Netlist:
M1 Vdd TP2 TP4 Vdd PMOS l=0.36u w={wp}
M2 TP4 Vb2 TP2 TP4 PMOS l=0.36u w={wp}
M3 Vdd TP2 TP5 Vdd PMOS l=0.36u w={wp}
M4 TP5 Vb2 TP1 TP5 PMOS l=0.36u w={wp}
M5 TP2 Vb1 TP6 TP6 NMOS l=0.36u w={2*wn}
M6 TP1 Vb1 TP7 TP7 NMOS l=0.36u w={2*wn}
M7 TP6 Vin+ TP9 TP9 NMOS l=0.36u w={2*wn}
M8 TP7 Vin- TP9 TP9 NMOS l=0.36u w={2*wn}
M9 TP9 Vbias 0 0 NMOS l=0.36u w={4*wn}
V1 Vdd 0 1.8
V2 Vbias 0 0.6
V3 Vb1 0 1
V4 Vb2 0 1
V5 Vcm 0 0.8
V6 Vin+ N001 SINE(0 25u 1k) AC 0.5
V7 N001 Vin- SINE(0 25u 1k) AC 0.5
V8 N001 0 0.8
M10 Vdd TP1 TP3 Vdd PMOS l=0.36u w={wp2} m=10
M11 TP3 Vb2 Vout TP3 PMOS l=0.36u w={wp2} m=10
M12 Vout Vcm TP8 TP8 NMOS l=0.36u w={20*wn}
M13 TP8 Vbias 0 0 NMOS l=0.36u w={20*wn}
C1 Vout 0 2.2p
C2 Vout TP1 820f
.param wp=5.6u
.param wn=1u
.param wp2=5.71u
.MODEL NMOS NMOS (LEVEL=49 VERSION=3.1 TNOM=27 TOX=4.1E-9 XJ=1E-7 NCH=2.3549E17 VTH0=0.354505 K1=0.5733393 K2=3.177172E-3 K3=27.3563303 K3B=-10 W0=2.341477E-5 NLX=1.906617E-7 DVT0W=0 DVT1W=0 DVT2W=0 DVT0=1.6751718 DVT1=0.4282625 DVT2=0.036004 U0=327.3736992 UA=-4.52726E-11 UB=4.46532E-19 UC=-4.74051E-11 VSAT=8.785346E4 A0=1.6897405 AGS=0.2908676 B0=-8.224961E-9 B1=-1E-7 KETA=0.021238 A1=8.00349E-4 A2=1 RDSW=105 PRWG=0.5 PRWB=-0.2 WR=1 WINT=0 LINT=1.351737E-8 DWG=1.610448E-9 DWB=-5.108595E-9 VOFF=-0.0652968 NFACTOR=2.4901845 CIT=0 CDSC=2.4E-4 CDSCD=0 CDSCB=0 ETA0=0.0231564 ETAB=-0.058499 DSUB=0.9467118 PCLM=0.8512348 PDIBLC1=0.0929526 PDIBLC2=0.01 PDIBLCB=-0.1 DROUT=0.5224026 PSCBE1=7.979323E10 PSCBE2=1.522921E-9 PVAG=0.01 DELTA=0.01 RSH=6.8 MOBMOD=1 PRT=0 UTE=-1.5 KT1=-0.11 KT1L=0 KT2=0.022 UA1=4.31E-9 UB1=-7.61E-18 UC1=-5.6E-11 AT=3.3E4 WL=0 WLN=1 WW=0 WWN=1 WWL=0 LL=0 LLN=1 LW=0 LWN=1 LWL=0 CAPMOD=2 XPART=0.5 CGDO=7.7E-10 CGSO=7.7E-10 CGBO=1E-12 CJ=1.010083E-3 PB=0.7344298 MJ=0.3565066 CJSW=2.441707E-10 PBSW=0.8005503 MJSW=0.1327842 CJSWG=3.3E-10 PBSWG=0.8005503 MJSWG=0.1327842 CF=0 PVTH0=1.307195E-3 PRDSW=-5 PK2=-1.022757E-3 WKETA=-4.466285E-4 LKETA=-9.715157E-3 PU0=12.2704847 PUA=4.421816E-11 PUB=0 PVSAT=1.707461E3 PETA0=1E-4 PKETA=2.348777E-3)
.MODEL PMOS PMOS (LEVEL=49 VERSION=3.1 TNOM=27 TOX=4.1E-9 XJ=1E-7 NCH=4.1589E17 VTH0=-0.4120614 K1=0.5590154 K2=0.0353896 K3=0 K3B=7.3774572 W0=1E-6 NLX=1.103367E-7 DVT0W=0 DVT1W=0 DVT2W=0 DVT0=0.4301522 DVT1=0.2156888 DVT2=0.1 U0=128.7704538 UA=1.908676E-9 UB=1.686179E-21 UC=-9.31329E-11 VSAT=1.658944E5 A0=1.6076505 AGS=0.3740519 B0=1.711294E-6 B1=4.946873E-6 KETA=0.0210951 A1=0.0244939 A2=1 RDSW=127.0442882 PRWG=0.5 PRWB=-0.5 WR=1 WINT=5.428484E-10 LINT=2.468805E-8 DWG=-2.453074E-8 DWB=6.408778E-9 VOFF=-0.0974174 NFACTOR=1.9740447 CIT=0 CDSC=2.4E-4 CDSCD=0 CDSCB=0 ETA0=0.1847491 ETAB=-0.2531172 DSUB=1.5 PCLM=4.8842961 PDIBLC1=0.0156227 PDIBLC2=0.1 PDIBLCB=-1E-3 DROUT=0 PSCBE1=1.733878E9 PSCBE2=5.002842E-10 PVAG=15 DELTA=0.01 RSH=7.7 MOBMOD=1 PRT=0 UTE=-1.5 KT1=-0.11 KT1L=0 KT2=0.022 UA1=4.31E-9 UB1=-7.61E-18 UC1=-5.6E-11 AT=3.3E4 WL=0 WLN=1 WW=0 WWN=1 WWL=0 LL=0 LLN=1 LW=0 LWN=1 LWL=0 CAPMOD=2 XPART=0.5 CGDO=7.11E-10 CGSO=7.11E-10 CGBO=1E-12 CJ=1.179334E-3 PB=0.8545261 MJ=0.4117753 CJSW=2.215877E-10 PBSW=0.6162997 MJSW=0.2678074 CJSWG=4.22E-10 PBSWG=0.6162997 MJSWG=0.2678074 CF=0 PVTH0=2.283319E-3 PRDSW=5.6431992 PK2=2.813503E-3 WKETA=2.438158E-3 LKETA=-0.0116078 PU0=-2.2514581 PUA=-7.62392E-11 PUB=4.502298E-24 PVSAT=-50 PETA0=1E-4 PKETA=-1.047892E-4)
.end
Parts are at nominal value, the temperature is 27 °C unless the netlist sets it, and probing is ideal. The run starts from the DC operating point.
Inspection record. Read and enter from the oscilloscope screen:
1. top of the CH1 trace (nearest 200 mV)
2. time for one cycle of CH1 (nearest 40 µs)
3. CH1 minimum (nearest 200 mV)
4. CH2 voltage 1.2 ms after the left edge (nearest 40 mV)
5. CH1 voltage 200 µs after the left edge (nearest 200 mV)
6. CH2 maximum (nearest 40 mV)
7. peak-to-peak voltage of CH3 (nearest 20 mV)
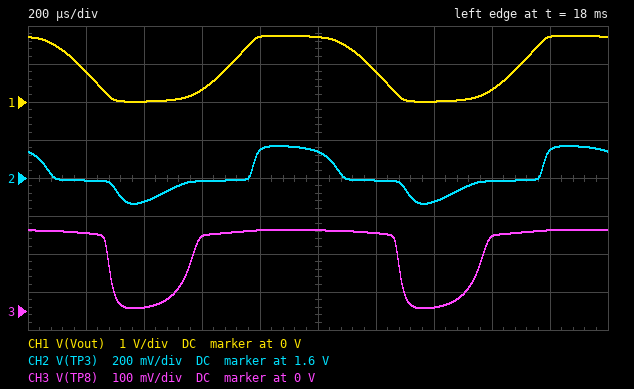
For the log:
1.8 V
1.00 ms
0 V
1.60 V
800 mV
1.76 V
200 mV
